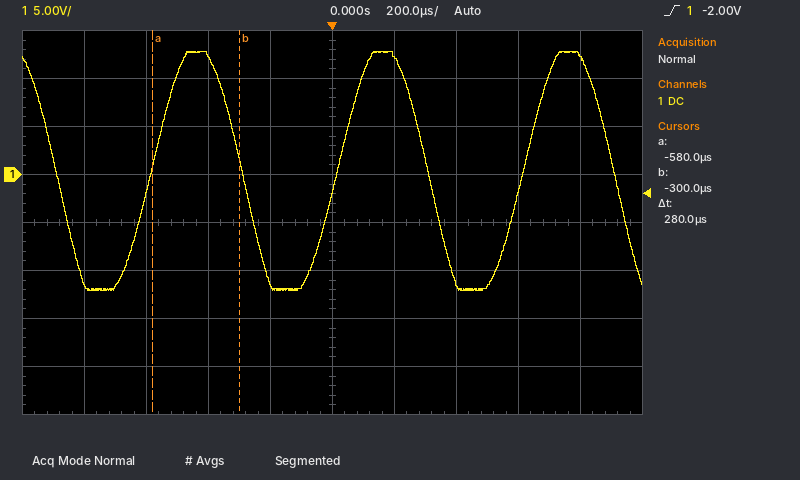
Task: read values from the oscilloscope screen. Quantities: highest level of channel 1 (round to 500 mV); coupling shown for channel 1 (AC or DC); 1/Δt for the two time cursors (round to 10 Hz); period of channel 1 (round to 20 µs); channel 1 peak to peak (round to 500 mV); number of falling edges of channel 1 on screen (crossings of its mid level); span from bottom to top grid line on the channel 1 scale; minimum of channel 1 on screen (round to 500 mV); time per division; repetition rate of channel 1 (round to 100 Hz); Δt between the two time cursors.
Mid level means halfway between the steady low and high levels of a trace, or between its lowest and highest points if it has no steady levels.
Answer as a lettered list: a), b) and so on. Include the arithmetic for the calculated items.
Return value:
a) 13.0 V
b) DC
c) 1 / 280 µs ≈ 3.57 kHz
d) 600 µs
e) 13.0 V − (-12.0 V) = 25.0 V
f) 4
g) 40 V
h) -12.0 V
i) 200 µs
j) 1 / 600 µs ≈ 1.7 kHz
k) 280 µs
